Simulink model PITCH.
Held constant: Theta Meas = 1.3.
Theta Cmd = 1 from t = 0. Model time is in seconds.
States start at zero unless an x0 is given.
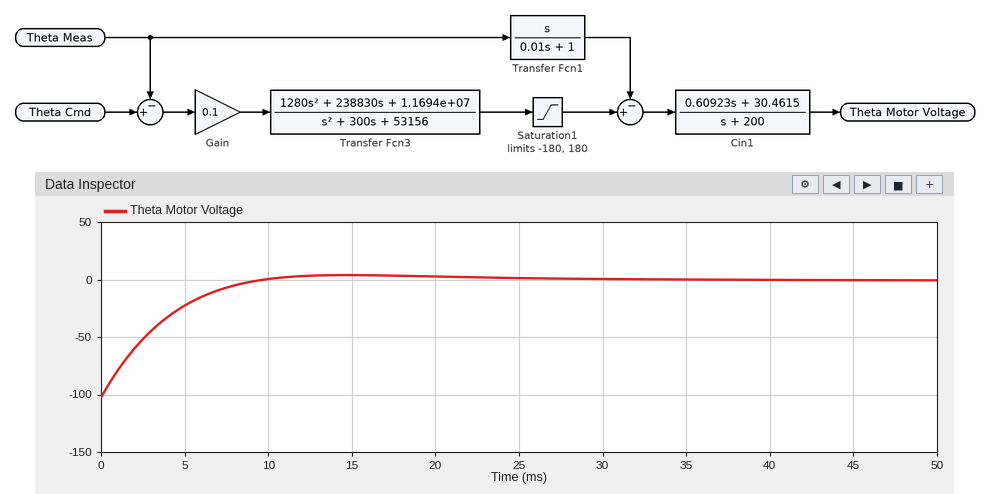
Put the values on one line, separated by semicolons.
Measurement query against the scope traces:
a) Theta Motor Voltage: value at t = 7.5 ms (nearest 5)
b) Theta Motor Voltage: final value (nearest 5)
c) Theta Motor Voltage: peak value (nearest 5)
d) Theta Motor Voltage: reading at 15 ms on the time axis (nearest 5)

-5; 0; 5; 5
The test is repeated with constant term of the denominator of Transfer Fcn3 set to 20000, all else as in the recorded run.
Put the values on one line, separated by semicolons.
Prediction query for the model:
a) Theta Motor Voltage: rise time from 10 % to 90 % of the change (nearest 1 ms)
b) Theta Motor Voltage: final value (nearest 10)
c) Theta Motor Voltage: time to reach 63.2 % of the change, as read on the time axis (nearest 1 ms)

7 ms; 0; 4 ms
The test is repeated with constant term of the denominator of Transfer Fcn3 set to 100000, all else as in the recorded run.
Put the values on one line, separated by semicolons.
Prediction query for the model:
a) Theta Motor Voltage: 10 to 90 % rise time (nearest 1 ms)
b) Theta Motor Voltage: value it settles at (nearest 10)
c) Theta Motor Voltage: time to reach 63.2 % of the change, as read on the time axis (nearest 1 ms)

6 ms; 0; 3 ms
